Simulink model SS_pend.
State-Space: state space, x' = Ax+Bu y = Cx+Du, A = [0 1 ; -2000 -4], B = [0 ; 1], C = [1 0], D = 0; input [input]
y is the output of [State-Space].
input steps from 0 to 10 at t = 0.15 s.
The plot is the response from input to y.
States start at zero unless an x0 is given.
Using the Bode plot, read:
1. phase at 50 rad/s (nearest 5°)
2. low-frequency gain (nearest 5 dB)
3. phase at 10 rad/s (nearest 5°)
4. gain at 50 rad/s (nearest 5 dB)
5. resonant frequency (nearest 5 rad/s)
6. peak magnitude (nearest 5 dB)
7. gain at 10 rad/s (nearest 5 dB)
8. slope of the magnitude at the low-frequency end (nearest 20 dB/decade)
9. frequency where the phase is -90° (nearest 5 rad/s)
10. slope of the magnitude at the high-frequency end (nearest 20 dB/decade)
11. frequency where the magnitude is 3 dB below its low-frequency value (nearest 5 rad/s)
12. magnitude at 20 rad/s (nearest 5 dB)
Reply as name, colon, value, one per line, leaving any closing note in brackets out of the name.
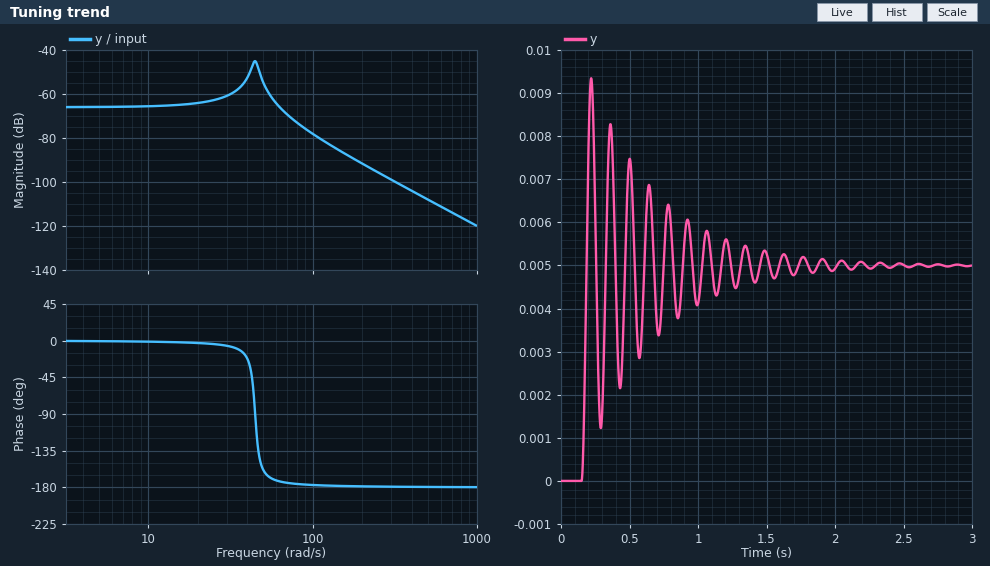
phase at 50 rad/s: -160°
low-frequency gain: -65 dB
phase at 10 rad/s: 0°
gain at 50 rad/s: -55 dB
resonant frequency: 45 rad/s
peak magnitude: -45 dB
gain at 10 rad/s: -65 dB
slope of the magnitude at the low-frequency end: 0 dB/decade
frequency where the phase is -90°: 45 rad/s
slope of the magnitude at the high-frequency end: -40 dB/decade
frequency where the magnitude is 3 dB below its low-frequency value: 70 rad/s
magnitude at 20 rad/s: -65 dB
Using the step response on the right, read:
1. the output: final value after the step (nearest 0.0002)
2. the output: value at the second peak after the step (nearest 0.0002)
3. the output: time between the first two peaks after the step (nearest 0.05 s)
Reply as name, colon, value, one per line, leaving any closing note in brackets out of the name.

the output: final value after the step: 0.0050
the output: value at the second peak after the step: 0.0082
the output: time between the first two peaks after the step: 0.15 s
